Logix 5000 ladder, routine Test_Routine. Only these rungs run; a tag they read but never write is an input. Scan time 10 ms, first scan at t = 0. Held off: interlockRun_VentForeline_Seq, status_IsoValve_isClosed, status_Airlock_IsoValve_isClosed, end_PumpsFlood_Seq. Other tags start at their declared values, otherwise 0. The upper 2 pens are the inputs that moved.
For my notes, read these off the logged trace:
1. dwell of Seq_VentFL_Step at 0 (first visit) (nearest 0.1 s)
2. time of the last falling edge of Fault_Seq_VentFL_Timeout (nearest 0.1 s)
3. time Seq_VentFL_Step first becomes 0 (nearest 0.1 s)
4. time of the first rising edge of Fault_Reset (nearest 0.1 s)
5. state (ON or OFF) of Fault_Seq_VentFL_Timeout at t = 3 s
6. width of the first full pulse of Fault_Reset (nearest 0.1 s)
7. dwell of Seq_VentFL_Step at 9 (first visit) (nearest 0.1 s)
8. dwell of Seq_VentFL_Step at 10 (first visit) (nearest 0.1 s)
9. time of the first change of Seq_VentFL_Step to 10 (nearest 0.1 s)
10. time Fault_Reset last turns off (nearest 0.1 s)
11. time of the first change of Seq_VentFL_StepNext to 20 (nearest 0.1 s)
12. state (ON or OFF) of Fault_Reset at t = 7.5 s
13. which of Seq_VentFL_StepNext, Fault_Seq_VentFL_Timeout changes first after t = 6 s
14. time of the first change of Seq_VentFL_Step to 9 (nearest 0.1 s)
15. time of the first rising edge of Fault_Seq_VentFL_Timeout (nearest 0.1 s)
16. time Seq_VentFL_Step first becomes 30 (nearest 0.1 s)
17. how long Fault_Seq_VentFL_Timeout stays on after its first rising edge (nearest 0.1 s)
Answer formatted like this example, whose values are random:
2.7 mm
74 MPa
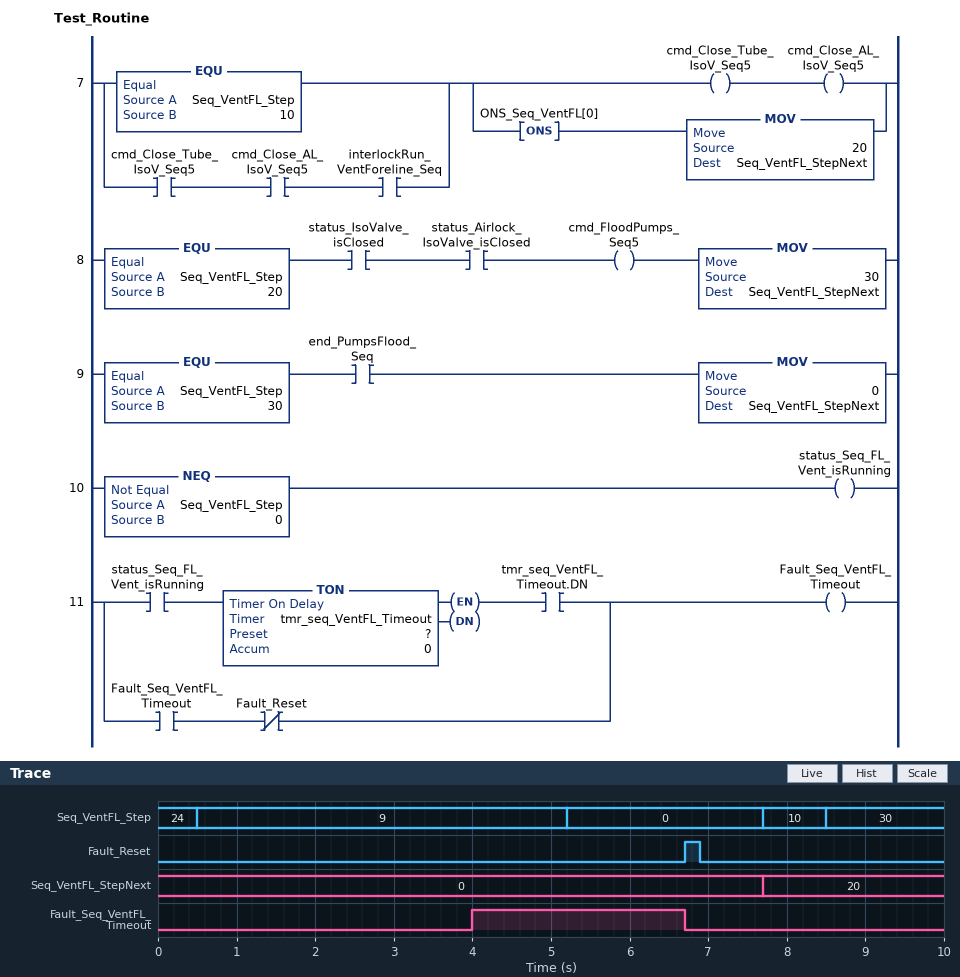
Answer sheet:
2.5 s
6.7 s
5.2 s
6.7 s
OFF
0.2 s
4.7 s
0.8 s
7.7 s
6.9 s
7.7 s
OFF
Fault_Seq_VentFL_Timeout
0.5 s
4.0 s
8.5 s
2.7 s
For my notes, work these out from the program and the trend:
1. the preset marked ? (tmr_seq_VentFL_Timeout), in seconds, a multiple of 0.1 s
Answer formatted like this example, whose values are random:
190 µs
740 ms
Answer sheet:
4.0 s
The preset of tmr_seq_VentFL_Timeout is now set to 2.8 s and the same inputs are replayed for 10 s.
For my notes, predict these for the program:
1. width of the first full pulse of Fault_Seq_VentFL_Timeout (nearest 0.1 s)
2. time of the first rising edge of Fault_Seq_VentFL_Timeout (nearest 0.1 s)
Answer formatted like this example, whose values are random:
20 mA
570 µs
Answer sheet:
3.9 s
2.8 s
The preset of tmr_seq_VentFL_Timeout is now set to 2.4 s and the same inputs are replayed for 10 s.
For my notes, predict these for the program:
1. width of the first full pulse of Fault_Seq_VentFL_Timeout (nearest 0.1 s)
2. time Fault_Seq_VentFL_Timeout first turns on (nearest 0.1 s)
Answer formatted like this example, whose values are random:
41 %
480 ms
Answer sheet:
4.3 s
2.4 s
